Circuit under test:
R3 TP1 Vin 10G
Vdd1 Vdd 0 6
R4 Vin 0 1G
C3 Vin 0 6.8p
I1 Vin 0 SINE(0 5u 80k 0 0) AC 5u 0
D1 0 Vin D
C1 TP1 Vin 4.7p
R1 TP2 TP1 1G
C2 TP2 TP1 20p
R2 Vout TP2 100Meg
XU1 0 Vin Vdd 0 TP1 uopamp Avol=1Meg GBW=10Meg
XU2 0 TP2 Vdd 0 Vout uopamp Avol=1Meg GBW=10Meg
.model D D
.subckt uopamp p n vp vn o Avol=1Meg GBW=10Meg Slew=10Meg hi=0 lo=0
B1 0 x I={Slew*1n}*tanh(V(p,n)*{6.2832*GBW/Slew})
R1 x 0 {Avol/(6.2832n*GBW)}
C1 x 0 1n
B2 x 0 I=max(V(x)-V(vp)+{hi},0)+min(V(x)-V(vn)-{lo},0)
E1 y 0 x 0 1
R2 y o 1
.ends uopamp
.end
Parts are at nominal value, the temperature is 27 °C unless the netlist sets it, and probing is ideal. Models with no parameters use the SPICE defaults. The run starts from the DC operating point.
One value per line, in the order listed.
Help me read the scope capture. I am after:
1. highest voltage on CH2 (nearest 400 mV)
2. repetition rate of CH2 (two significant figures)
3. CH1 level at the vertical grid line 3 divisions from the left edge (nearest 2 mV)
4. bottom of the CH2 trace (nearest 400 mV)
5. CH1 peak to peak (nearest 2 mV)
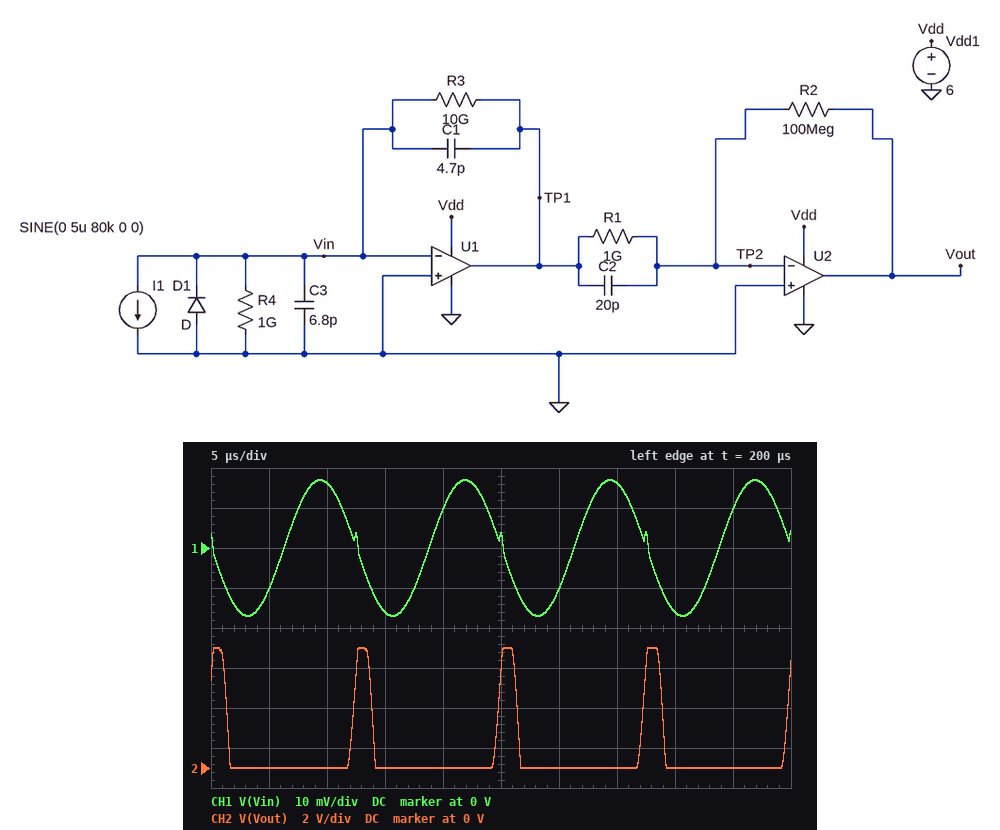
6.0 V
80 kHz
-16 mV
0 V
34 mV
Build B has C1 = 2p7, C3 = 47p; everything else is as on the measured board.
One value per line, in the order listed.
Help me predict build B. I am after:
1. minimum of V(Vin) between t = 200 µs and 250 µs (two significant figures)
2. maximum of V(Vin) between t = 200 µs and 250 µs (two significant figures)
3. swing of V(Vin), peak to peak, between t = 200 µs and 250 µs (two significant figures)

-73 mV
29 mV
100 mV
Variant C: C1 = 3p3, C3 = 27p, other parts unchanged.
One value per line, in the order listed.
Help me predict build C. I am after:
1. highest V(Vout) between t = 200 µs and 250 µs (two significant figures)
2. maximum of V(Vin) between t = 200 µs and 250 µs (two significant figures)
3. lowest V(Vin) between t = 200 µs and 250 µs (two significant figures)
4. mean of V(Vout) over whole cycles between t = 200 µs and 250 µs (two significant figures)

6.0 V
24 mV
-24 mV
800 mV
